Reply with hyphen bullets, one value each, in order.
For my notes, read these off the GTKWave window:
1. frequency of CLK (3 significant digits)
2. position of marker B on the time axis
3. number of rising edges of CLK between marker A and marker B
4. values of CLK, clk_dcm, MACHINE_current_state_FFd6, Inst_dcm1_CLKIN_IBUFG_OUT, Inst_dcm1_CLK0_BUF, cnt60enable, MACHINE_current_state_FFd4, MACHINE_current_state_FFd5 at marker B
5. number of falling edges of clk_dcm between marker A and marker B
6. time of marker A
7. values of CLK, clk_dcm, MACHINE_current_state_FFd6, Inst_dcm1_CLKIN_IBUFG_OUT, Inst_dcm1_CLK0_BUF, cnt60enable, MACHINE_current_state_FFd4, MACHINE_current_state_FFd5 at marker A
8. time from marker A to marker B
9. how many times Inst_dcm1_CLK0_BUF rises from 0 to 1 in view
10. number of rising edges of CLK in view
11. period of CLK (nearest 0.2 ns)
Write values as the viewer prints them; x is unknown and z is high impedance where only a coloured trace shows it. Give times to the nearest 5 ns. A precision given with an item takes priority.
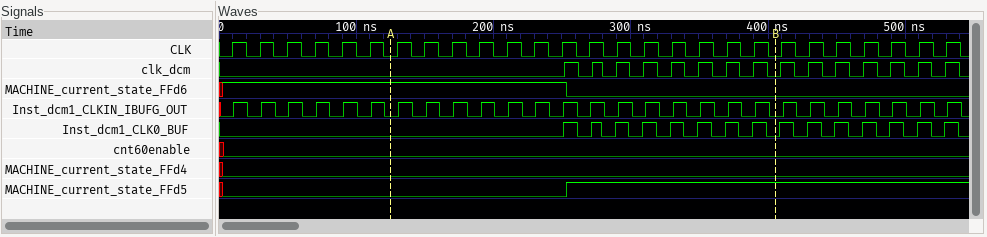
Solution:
- 50.0 MHz
- 405 ns
- 14
- CLK=0, clk_dcm=0, MACHINE_current_state_FFd6=0, Inst_dcm1_CLKIN_IBUFG_OUT=0, Inst_dcm1_CLK0_BUF=0, cnt60enable=0, MACHINE_current_state_FFd4=0, MACHINE_current_state_FFd5=1
- 8
- 125 ns
- CLK=0, clk_dcm=0, MACHINE_current_state_FFd6=1, Inst_dcm1_CLKIN_IBUFG_OUT=0, Inst_dcm1_CLK0_BUF=0, cnt60enable=0, MACHINE_current_state_FFd4=0, MACHINE_current_state_FFd5=0
- 280 ns
- 15
- 27
- 20 ns
